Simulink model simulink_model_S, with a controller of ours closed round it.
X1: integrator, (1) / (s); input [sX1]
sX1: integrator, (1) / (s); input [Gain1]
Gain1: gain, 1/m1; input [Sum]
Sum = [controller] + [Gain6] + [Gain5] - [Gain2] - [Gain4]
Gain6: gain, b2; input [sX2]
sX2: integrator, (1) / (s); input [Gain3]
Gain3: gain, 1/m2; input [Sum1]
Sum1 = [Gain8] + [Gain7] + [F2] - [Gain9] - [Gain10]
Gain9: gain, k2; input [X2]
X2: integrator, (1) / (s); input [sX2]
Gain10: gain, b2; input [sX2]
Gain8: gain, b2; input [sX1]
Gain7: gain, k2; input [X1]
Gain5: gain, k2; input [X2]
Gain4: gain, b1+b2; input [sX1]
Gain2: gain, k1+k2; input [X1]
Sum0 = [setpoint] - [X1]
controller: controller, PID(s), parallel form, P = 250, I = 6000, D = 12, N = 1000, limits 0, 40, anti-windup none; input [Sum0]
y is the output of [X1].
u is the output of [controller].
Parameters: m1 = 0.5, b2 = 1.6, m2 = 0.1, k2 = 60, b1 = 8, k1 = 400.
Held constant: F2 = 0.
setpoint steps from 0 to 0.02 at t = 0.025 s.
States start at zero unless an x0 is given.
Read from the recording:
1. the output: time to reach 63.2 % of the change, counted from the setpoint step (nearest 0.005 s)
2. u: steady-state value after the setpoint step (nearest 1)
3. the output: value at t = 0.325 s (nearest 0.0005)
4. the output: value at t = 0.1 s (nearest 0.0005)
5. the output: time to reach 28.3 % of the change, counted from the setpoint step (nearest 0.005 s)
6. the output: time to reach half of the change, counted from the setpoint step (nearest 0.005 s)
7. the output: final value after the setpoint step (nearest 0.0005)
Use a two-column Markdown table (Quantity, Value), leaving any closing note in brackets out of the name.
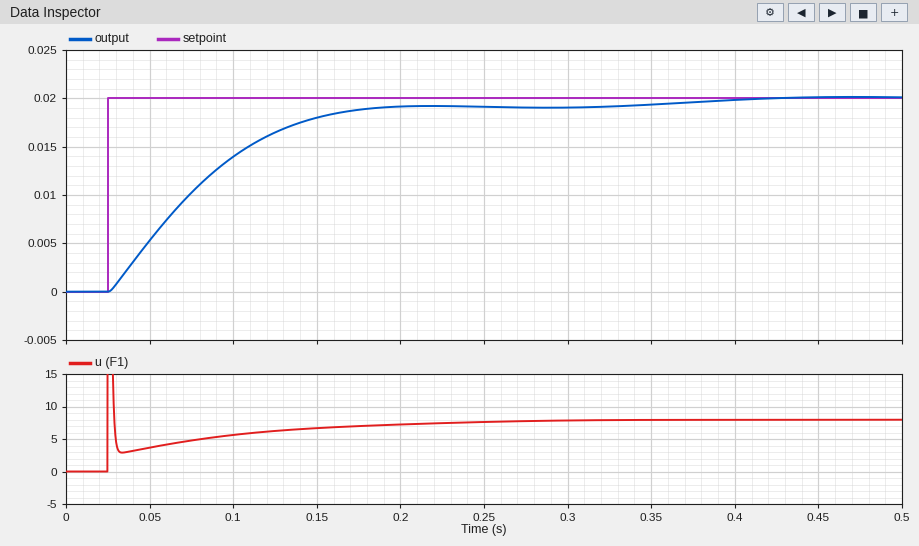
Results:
| Quantity | Value |
|---|---|
| the output: time to reach 63.2 % of the change, counted from the setpoint step | 0.065 s |
| u: steady-state value after the setpoint step | 8 |
| the output: value at t = 0.325 s | 0.0190 |
| the output: value at t = 0.1 s | 0.0140 |
| the output: time to reach 28.3 % of the change, counted from the setpoint step | 0.025 s |
| the output: time to reach half of the change, counted from the setpoint step | 0.050 s |
| the output: final value after the setpoint step | 0.0200 |
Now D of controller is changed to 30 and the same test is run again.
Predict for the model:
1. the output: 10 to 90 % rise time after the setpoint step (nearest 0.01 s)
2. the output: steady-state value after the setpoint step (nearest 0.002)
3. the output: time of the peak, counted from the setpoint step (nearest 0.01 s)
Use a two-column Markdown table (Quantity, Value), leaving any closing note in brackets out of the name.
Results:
| Quantity | Value |
|---|---|
| the output: 10 to 90 % rise time after the setpoint step | 0.14 s |
| the output: steady-state value after the setpoint step | 0.020 |
| the output: time of the peak, counted from the setpoint step | 0.26 s |
